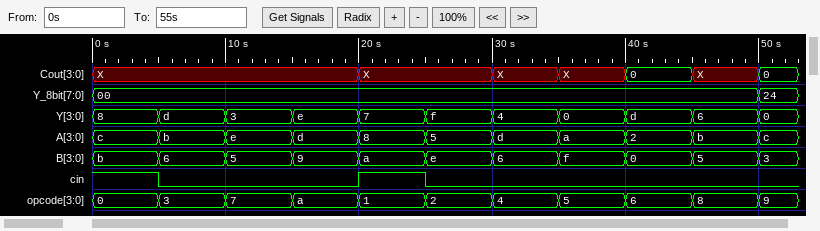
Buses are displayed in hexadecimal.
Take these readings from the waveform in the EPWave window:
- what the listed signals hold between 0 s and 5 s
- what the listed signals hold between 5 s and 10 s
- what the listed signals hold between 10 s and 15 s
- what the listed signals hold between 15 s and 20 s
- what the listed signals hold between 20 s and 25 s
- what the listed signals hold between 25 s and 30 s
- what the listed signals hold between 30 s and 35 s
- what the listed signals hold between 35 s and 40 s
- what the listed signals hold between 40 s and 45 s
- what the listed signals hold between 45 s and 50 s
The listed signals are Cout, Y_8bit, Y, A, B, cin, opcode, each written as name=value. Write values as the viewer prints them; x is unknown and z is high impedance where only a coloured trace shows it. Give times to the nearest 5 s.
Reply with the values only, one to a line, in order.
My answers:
Cout=X, Y_8bit=00, Y=8, A=c, B=b, cin=1, opcode=0
Cout=X, Y_8bit=00, Y=d, A=b, B=6, cin=0, opcode=3
Cout=X, Y_8bit=00, Y=3, A=e, B=5, cin=0, opcode=7
Cout=X, Y_8bit=00, Y=e, A=d, B=9, cin=0, opcode=a
Cout=X, Y_8bit=00, Y=7, A=8, B=a, cin=1, opcode=1
Cout=X, Y_8bit=00, Y=f, A=5, B=e, cin=0, opcode=2
Cout=X, Y_8bit=00, Y=4, A=d, B=6, cin=0, opcode=4
Cout=X, Y_8bit=00, Y=0, A=a, B=f, cin=0, opcode=5
Cout=0, Y_8bit=00, Y=d, A=2, B=0, cin=0, opcode=6
Cout=X, Y_8bit=00, Y=6, A=b, B=5, cin=0, opcode=8
